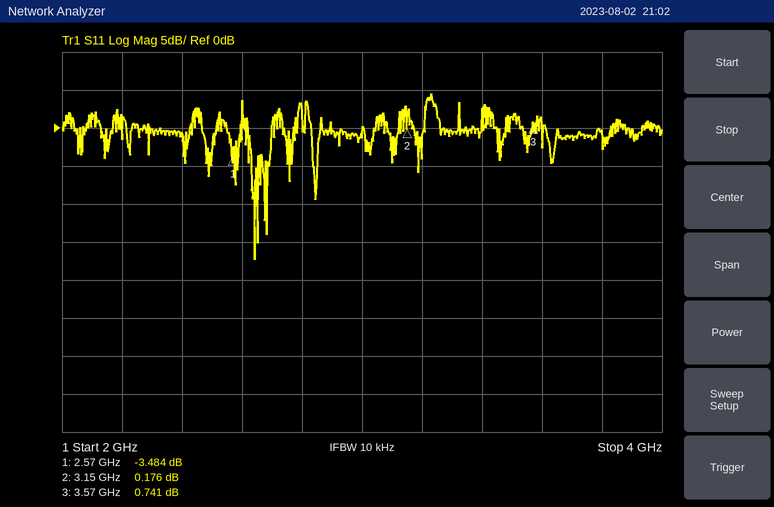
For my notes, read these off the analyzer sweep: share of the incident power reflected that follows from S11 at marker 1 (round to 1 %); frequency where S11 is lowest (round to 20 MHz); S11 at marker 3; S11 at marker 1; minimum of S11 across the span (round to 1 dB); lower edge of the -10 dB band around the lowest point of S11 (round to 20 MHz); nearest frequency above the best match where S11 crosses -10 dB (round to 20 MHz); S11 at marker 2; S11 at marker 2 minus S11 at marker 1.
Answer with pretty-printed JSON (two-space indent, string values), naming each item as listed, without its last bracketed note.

{
  "share of the incident power reflected that follows from S11 at marker 1": "45 %",
  "frequency where S11 is lowest": "2.64 GHz",
  "S11 at marker 3": "0.741 dB",
  "S11 at marker 1": "-3.484 dB",
  "minimum of S11 across the span": "-17 dB",
  "lower edge of the -10 dB band around the lowest point of S11": "2.64 GHz",
  "nearest frequency above the best match where S11 crosses -10 dB": "2.64 GHz",
  "S11 at marker 2": "0.176 dB",
  "S11 at marker 2 minus S11 at marker 1": "3.660 dB"
}
